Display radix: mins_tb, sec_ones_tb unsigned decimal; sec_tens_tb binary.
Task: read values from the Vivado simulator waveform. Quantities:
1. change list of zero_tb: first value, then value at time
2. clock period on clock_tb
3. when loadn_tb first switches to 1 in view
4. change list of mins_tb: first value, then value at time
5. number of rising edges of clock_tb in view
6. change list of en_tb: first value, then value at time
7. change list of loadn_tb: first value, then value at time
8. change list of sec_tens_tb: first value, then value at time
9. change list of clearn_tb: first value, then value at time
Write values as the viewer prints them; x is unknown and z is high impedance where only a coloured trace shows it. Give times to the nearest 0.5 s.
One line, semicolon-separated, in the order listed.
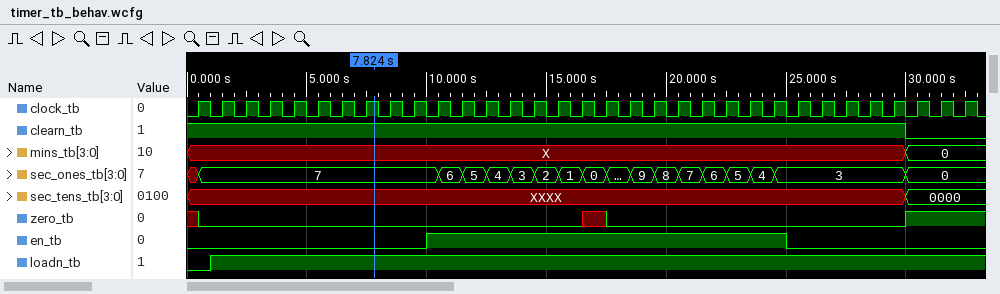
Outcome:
x, 0 at 0.5 s, x at 16.5 s, 0 at 17.5 s, 1 at 30 s; 1 s; 1 s; X, 0 at 30 s; 33; 0, 1 at 10 s, 0 at 25 s; 0, 1 at 1 s; XXXX, 0000 at 30 s; 1, 0 at 30 s
